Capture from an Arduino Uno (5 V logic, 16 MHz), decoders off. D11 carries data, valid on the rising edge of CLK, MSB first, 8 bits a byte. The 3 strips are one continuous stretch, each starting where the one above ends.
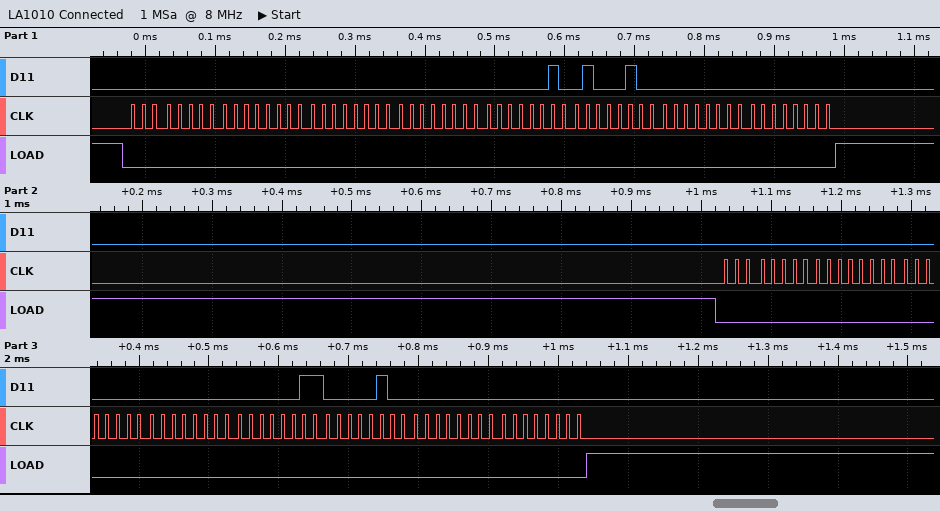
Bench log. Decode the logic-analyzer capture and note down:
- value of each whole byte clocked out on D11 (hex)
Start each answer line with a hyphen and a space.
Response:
- 00 00 00 00 02 44 00 00 00 00 00 00 03 04 00 00
